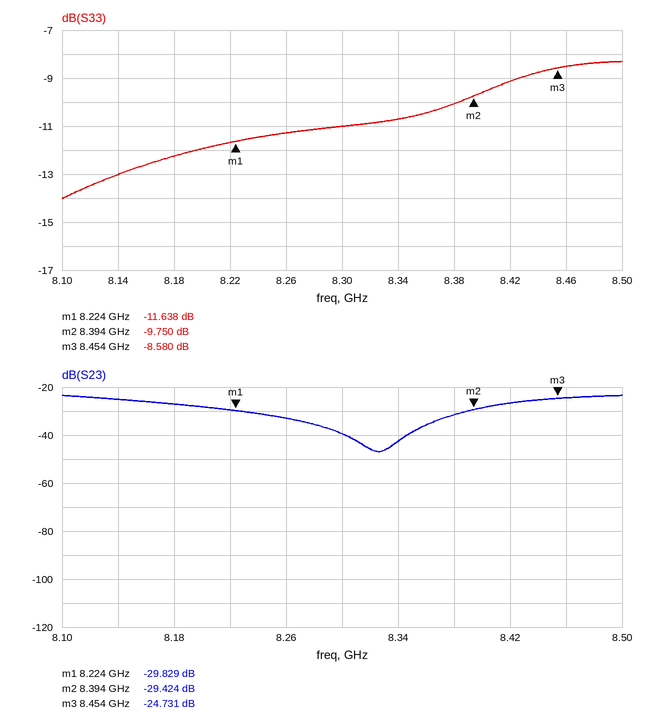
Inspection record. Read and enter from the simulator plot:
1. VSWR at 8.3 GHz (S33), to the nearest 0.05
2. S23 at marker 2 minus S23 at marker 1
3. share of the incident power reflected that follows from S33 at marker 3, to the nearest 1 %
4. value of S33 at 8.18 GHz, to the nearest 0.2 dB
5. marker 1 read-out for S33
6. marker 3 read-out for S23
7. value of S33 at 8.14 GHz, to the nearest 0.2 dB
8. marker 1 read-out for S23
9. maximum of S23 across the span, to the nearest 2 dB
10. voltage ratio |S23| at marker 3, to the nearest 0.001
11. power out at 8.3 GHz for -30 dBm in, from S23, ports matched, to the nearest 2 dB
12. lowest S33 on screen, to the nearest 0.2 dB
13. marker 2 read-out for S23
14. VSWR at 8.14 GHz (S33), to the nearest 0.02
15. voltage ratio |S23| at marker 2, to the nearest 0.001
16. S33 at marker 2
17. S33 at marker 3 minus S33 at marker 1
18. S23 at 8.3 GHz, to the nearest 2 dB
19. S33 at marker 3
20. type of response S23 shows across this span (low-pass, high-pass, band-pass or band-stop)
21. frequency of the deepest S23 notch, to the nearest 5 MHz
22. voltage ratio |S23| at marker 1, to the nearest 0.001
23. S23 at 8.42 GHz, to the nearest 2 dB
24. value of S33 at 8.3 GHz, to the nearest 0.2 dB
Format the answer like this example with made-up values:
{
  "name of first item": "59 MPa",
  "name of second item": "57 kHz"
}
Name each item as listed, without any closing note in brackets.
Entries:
{
  "VSWR at 8.3 GHz (S33), to the nearest 0.05": "1.80",
  "S23 at marker 2 minus S23 at marker 1": "0.405 dB",
  "share of the incident power reflected that follows from S33 at marker 3, to the nearest 1 %": "14 %",
  "value of S33 at 8.18 GHz, to the nearest 0.2 dB": "-12.2 dB",
  "marker 1 read-out for S33": "-11.638 dB",
  "marker 3 read-out for S23": "-24.731 dB",
  "value of S33 at 8.14 GHz, to the nearest 0.2 dB": "-13.0 dB",
  "marker 1 read-out for S23": "-29.829 dB",
  "maximum of S23 across the span, to the nearest 2 dB": "-24 dB",
  "voltage ratio |S23| at marker 3, to the nearest 0.001": "0.058",
  "power out at 8.3 GHz for -30 dBm in, from S23, ports matched, to the nearest 2 dB": "-70 dBm",
  "lowest S33 on screen, to the nearest 0.2 dB": "-14.0 dB",
  "marker 2 read-out for S23": "-29.424 dB",
  "VSWR at 8.14 GHz (S33), to the nearest 0.02": "1.58",
  "voltage ratio |S23| at marker 2, to the nearest 0.001": "0.034",
  "S33 at marker 2": "-9.750 dB",
  "S33 at marker 3 minus S33 at marker 1": "3.058 dB",
  "S23 at 8.3 GHz, to the nearest 2 dB": "-40 dB",
  "S33 at marker 3": "-8.580 dB",
  "type of response S23 shows across this span": "band-stop",
  "frequency of the deepest S23 notch, to the nearest 5 MHz": "8.325 GHz",
  "voltage ratio |S23| at marker 1, to the nearest 0.001": "0.032",
  "S23 at 8.42 GHz, to the nearest 2 dB": "-26 dB",
  "value of S33 at 8.3 GHz, to the nearest 0.2 dB": "-11.0 dB"
}
